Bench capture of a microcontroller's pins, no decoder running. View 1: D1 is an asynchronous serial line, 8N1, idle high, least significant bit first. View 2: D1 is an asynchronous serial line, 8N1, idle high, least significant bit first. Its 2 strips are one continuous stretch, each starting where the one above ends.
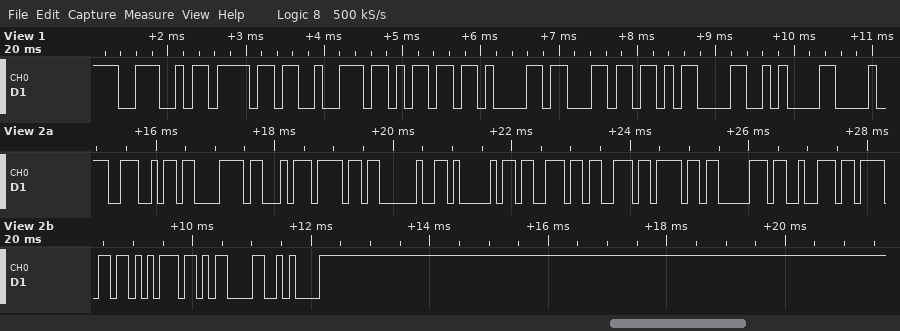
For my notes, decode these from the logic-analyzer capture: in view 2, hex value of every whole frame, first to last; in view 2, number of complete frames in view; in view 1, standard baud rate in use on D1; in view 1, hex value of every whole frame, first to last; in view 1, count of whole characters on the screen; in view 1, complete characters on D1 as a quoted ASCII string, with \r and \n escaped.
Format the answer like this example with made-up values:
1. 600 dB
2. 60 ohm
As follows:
1. 4E C3 A3 6F 20 41 73 73 6F 70 72 6F 75 0D 0A
2. 15
3. 9600 baud
4. 4E 6F 72 6D 61 6C 0D 0A
5. 8
6. "Normal\r\n"
